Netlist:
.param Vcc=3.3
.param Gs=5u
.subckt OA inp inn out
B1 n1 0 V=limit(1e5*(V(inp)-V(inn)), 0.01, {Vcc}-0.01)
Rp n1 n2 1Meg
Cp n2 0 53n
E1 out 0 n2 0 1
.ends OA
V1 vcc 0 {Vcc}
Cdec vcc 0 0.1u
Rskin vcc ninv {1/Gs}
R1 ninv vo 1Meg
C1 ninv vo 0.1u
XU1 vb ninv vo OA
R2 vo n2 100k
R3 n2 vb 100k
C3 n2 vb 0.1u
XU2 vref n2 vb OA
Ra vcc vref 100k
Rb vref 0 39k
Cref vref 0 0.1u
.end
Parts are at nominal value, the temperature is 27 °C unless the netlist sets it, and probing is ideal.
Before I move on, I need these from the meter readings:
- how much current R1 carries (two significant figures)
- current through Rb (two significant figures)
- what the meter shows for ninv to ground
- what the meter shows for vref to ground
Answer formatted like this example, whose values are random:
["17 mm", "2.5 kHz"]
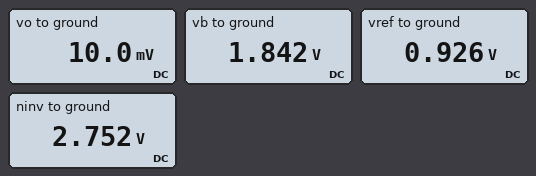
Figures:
["2.7 µA", "24 µA", "2.752 V", "0.926 V"]
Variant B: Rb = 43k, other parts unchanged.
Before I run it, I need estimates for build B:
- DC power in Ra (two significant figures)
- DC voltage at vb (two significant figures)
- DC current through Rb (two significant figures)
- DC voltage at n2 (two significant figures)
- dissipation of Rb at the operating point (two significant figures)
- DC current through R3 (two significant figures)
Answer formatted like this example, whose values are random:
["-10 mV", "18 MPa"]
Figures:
["53 µW", "2.0 V", "23 µA", "990 mV", "23 µW", "9.8 µA"]
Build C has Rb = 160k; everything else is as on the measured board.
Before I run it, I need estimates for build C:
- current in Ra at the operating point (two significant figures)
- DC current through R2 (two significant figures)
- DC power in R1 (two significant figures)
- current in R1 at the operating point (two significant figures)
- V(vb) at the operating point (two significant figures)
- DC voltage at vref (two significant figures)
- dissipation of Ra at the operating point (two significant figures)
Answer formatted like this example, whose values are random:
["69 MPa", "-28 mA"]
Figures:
["13 µA", "9.1 µA", "3.3 µW", "1.8 µA", "2.9 V", "2.0 V", "16 µW"]
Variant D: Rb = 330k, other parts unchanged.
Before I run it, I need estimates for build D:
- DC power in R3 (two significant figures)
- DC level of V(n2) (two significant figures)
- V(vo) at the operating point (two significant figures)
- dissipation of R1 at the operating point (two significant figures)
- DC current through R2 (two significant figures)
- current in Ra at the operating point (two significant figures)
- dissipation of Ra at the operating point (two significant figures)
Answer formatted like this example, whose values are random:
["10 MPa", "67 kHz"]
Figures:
["3.0 µW", "2.5 V", "2.0 V", "1.2 µW", "5.5 µA", "7.7 µA", "5.9 µW"]
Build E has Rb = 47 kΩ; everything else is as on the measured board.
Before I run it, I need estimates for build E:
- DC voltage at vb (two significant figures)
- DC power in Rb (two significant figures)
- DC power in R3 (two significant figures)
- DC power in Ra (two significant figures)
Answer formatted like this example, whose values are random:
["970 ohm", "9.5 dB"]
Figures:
["2.1 V", "24 µW", "11 µW", "50 µW"]
